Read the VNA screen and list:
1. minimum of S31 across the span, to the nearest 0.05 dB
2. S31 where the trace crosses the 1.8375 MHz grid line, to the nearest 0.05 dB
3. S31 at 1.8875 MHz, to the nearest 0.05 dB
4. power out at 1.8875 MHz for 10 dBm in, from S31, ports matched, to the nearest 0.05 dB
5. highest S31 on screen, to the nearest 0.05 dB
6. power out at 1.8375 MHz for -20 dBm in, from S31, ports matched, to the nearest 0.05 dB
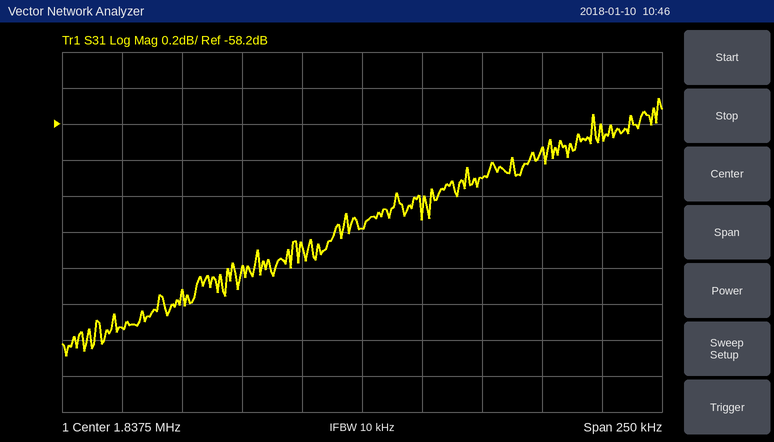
-59.50 dB
-58.80 dB
-58.50 dB
-48.50 dBm
-58.05 dB
-78.80 dBm
